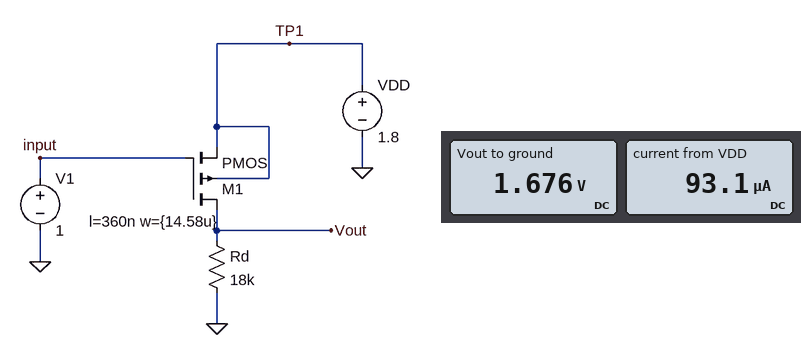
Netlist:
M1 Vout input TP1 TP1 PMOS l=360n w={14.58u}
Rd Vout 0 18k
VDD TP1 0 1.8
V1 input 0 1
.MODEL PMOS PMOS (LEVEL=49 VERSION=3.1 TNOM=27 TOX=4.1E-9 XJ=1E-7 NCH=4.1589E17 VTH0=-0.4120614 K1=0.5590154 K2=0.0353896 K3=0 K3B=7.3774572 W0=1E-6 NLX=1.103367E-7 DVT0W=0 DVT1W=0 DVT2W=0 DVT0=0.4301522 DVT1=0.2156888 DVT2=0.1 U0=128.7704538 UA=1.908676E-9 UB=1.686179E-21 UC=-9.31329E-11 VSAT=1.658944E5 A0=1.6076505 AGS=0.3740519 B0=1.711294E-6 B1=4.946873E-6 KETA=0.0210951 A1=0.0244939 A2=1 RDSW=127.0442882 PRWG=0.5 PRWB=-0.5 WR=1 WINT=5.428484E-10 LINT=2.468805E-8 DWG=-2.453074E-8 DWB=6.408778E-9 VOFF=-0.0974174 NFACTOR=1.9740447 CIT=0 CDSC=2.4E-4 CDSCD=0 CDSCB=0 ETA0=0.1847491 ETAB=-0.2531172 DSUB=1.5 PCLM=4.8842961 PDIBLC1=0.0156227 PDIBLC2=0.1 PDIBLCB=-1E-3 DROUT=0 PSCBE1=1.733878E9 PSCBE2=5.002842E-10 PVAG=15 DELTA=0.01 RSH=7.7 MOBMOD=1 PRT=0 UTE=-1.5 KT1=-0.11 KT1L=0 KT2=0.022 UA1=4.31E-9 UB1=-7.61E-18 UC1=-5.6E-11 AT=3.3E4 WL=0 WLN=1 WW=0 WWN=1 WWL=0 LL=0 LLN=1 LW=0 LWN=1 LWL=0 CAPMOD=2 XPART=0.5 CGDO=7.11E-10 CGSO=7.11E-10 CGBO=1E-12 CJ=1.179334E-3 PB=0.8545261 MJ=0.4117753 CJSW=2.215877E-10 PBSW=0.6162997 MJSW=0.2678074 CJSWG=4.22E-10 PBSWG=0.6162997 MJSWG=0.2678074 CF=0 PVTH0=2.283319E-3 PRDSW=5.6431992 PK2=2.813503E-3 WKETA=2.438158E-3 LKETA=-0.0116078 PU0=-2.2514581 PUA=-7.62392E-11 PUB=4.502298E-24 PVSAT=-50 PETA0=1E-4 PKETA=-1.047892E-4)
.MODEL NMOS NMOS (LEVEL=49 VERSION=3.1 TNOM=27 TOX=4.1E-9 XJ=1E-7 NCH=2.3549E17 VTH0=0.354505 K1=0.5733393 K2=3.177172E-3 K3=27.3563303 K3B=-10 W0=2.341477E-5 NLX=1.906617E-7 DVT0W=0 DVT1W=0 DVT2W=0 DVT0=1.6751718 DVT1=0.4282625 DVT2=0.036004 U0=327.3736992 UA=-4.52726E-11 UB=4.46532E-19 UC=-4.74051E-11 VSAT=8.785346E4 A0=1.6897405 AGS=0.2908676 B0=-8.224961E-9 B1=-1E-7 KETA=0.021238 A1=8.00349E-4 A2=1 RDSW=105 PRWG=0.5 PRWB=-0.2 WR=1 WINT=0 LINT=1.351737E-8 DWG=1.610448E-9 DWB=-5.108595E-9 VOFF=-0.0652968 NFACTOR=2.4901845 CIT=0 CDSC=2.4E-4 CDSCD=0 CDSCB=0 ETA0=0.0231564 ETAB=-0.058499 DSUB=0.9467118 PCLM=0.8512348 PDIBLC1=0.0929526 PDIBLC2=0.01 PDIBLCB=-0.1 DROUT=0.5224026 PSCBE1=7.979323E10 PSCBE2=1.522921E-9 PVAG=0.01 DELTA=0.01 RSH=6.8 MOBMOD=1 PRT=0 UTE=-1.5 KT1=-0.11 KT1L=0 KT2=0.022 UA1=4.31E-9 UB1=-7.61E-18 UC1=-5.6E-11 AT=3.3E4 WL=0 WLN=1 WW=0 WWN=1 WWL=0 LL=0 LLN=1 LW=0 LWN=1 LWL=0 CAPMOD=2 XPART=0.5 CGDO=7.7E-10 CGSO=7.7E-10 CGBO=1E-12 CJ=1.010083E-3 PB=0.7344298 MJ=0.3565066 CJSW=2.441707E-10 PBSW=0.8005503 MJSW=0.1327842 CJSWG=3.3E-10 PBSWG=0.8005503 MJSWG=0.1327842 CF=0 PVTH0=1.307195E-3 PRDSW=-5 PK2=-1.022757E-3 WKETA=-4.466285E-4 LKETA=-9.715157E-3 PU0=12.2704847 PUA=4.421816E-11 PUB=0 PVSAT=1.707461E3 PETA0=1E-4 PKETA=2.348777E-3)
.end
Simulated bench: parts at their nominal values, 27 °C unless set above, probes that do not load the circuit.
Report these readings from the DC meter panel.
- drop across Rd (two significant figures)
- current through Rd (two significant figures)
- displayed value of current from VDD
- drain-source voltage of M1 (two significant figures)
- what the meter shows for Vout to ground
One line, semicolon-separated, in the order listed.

1.7 V; 93 µA; 93.1 µA; -120 mV; 1.676 V
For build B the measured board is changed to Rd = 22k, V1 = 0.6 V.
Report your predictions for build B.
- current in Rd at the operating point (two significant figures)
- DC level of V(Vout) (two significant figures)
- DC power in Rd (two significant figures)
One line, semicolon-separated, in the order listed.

80 µA; 1.8 V; 140 µW
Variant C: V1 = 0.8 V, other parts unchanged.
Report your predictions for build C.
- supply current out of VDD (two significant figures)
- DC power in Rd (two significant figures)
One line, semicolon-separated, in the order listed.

96 µA; 170 µW
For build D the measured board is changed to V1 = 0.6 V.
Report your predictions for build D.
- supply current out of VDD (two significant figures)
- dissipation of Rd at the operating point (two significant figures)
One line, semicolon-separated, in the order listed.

97 µA; 170 µW
